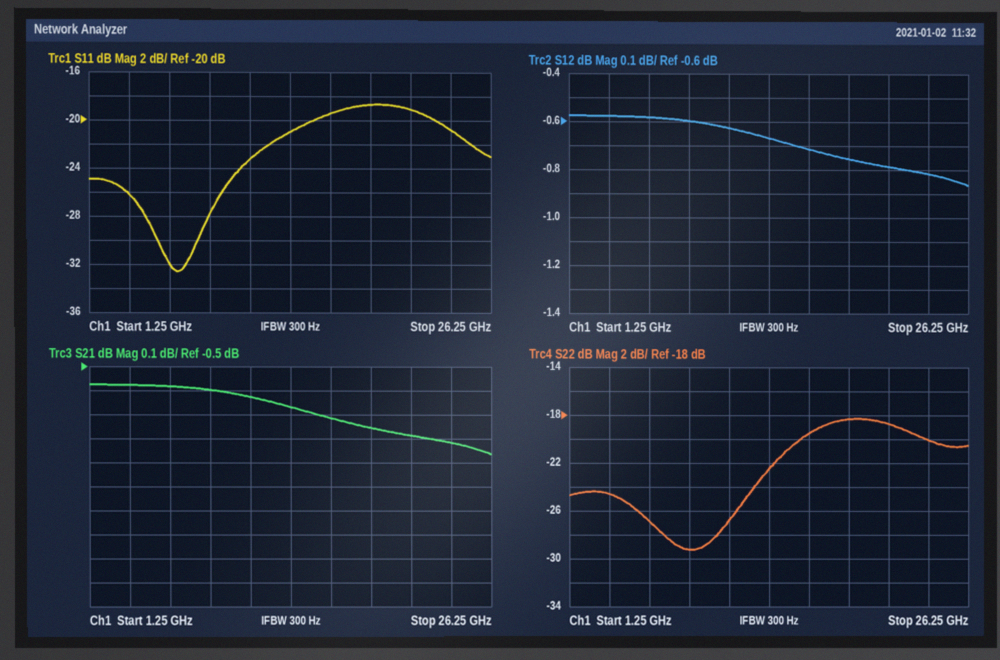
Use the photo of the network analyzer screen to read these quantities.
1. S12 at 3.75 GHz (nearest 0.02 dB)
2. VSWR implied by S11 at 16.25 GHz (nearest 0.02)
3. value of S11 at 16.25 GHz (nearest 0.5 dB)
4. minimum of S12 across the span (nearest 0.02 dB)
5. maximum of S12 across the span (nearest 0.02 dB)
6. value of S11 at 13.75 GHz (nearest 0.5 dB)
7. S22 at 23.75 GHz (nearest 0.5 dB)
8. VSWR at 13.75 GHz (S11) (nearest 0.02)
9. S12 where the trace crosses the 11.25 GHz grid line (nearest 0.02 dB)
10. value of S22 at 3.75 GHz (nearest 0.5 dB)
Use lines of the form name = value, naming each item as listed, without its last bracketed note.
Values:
S12 at 3.75 GHz = -0.58 dB
VSWR implied by S11 at 16.25 GHz = 1.24
value of S11 at 16.25 GHz = -19.5 dB
minimum of S12 across the span = -0.86 dB
maximum of S12 across the span = -0.58 dB
value of S11 at 13.75 GHz = -21.0 dB
S22 at 23.75 GHz = -20.0 dB
VSWR at 13.75 GHz (S11) = 1.20
S12 where the trace crosses the 11.25 GHz grid line = -0.62 dB
value of S22 at 3.75 GHz = -24.5 dB
